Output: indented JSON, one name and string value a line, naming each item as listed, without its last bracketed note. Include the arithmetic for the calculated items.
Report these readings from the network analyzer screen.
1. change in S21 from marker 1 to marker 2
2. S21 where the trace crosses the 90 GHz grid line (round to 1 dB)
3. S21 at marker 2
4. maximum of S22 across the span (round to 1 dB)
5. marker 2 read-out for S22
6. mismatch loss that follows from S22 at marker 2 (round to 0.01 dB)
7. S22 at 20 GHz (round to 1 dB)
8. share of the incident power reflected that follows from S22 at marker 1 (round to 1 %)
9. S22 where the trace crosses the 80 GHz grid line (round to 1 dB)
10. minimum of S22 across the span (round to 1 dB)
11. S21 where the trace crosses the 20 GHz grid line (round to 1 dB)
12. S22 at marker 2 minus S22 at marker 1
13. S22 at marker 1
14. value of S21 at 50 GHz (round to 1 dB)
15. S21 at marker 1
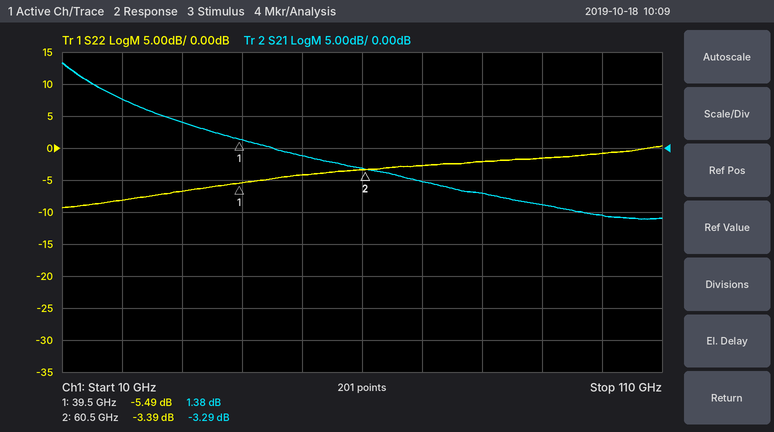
{
  "change in S21 from marker 1 to marker 2": "-3.29 − (1.38) = -4.67 dB",
  "S21 where the trace crosses the 90 GHz grid line": "-9 dB",
  "S21 at marker 2": "-3.29 dB",
  "maximum of S22 across the span": "0 dB",
  "marker 2 read-out for S22": "-3.39 dB",
  "mismatch loss that follows from S22 at marker 2": "−10 log10(1 − 10^(-3.39/10)) ≈ 2.66 dB",
  "S22 at 20 GHz": "-8 dB",
  "share of the incident power reflected that follows from S22 at marker 1": "10^(-5.49/10) ≈ 28 %",
  "S22 where the trace crosses the 80 GHz grid line": "-2 dB",
  "minimum of S22 across the span": "-9 dB",
  "S21 where the trace crosses the 20 GHz grid line": "8 dB",
  "S22 at marker 2 minus S22 at marker 1": "-3.39 − (-5.49) = 2.10 dB",
  "S22 at marker 1": "-5.49 dB",
  "value of S21 at 50 GHz": "-1 dB",
  "S21 at marker 1": "1.38 dB"
}
